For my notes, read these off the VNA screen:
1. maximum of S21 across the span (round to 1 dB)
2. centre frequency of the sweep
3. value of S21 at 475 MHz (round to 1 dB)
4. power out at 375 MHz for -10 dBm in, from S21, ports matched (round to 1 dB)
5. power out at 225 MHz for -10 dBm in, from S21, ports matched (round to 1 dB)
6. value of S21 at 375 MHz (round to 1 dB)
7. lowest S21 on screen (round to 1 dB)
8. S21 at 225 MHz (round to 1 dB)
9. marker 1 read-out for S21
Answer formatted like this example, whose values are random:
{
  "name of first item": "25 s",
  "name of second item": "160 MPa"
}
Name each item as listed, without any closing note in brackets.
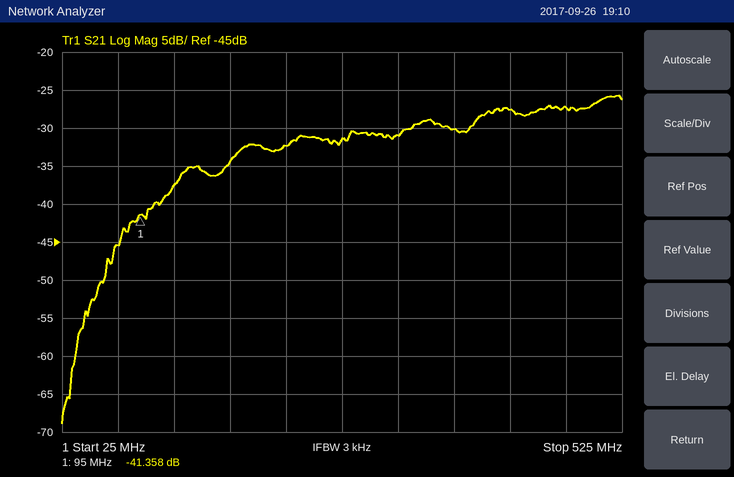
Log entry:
{
  "maximum of S21 across the span": "-26 dB",
  "centre frequency of the sweep": "275 MHz",
  "value of S21 at 475 MHz": "-27 dB",
  "power out at 375 MHz for -10 dBm in, from S21, ports matched": "-40 dBm",
  "power out at 225 MHz for -10 dBm in, from S21, ports matched": "-42 dBm",
  "value of S21 at 375 MHz": "-30 dB",
  "lowest S21 on screen": "-69 dB",
  "S21 at 225 MHz": "-32 dB",
  "marker 1 read-out for S21": "-41.358 dB"
}
